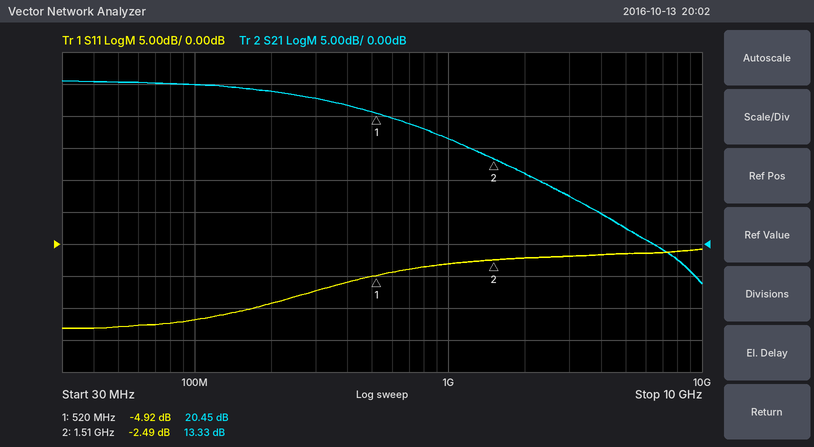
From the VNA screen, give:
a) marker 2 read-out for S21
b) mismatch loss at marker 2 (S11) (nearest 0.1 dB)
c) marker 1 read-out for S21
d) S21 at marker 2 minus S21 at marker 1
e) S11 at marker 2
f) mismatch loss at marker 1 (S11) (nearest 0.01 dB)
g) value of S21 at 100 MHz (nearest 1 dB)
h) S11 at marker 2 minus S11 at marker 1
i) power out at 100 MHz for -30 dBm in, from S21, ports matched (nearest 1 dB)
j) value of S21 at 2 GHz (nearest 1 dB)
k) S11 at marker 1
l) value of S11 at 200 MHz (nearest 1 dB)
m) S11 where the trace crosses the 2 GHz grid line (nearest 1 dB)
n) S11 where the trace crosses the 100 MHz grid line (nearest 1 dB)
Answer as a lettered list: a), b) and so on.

a) 13.33 dB
b) 3.6 dB
c) 20.45 dB
d) -7.12 dB
e) -2.49 dB
f) 1.69 dB
g) 25 dB
h) 2.43 dB
i) -5 dBm
j) 11 dB
k) -4.92 dB
l) -9 dB
m) -2 dB
n) -12 dB
